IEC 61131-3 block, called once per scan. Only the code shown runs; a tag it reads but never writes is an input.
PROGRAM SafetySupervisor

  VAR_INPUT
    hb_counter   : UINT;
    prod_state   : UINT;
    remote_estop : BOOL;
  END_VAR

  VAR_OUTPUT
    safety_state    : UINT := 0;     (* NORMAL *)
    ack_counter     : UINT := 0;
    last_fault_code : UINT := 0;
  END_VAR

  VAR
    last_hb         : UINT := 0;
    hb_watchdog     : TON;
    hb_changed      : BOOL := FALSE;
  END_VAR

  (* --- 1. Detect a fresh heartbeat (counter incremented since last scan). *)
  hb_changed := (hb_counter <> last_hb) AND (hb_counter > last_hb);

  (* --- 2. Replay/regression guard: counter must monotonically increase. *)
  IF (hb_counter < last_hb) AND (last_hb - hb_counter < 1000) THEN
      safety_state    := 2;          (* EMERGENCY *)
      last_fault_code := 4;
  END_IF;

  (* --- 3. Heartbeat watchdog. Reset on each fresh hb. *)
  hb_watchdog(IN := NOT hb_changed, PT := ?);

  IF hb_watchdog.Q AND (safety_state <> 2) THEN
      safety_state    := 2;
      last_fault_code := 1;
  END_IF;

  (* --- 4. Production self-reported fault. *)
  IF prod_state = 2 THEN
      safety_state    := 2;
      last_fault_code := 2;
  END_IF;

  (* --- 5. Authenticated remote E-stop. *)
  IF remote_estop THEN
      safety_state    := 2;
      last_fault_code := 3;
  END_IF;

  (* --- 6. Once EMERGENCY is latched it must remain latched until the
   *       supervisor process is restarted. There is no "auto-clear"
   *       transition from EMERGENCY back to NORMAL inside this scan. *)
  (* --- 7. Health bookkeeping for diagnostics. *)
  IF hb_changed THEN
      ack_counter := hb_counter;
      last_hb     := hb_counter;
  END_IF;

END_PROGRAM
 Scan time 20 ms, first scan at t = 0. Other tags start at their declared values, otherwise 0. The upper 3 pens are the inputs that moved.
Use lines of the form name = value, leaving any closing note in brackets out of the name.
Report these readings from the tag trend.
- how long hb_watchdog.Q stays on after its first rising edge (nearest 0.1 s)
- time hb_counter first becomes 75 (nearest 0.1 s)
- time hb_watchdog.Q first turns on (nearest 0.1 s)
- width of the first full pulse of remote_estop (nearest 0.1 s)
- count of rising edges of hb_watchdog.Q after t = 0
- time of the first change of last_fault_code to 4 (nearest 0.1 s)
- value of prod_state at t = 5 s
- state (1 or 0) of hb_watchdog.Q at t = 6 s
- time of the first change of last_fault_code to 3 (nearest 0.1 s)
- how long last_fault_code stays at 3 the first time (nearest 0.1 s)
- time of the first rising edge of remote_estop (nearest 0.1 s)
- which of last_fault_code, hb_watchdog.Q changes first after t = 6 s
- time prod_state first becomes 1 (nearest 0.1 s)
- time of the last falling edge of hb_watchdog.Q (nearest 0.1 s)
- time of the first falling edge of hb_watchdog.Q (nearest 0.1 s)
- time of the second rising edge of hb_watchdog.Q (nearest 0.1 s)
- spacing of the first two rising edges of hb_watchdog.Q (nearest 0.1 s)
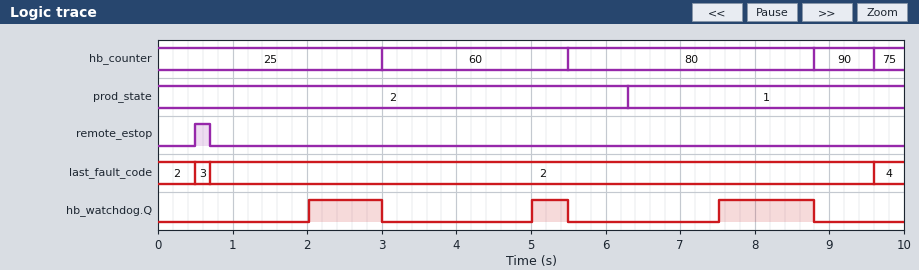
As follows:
how long hb_watchdog.Q stays on after its first rising edge = 1.0 s
time hb_counter first becomes 75 = 9.6 s
time hb_watchdog.Q first turns on = 2.0 s
width of the first full pulse of remote_estop = 0.2 s
count of rising edges of hb_watchdog.Q after t = 0 = 3
time of the first change of last_fault_code to 4 = 9.6 s
value of prod_state at t = 5 s = 2
state (1 or 0) of hb_watchdog.Q at t = 6 s = 0
time of the first change of last_fault_code to 3 = 0.5 s
how long last_fault_code stays at 3 the first time = 0.2 s
time of the first rising edge of remote_estop = 0.5 s
which of last_fault_code, hb_watchdog.Q changes first after t = 6 s = hb_watchdog.Q
time prod_state first becomes 1 = 6.3 s
time of the last falling edge of hb_watchdog.Q = 8.8 s
time of the first falling edge of hb_watchdog.Q = 3.0 s
time of the second rising edge of hb_watchdog.Q = 5.0 s
spacing of the first two rising edges of hb_watchdog.Q = 3.0 s
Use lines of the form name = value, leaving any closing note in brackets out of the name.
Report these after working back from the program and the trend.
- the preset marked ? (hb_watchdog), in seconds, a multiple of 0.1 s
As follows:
the preset marked ? (hb_watchdog), in seconds, a multiple of 0.1 s = 2.0 s
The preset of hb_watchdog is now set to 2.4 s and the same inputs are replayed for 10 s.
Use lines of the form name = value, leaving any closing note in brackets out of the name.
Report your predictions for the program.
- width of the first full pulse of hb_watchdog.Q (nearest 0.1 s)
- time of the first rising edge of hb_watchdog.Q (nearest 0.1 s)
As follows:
width of the first full pulse of hb_watchdog.Q = 0.6 s
time of the first rising edge of hb_watchdog.Q = 2.4 s
